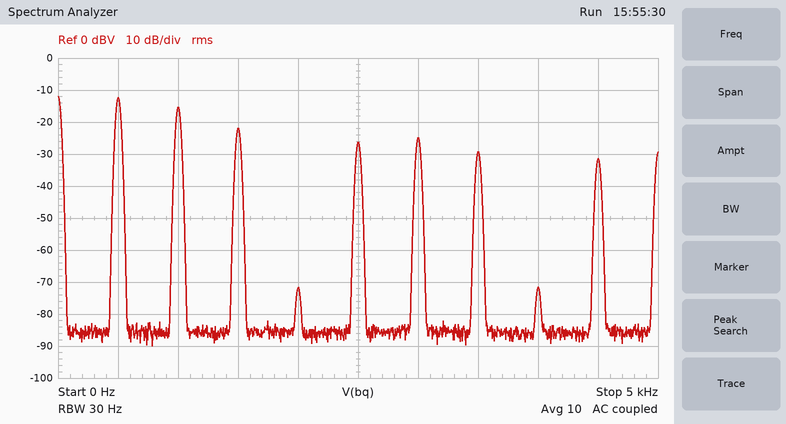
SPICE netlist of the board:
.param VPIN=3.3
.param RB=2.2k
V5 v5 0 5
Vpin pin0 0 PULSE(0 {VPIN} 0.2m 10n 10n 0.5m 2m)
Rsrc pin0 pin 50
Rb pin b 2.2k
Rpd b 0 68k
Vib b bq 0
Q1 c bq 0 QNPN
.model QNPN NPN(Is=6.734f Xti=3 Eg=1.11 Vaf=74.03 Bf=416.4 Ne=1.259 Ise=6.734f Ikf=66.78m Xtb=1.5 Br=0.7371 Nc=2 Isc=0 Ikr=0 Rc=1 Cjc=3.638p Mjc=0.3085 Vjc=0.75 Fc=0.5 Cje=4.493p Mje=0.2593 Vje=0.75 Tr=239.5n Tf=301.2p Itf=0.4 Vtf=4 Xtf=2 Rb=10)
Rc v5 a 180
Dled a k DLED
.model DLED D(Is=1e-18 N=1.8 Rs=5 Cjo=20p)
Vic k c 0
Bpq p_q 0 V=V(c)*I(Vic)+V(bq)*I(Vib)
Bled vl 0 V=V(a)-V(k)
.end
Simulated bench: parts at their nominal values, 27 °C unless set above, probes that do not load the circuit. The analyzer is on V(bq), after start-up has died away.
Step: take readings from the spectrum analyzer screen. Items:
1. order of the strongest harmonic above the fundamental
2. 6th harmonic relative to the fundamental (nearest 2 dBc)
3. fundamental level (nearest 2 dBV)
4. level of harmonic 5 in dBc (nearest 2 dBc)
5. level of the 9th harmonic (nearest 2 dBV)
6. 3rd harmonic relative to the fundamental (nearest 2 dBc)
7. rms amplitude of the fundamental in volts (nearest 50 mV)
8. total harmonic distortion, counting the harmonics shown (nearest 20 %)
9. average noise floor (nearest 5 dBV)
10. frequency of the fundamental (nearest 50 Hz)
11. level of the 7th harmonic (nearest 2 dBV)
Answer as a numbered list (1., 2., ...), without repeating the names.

1. 2
2. -12 dBc
3. -12 dBV
4. -14 dBc
5. -32 dBV
6. -10 dBc
7. 250 mV
8. 80 %
9. -85 dBV
10. 500 Hz
11. -30 dBV
